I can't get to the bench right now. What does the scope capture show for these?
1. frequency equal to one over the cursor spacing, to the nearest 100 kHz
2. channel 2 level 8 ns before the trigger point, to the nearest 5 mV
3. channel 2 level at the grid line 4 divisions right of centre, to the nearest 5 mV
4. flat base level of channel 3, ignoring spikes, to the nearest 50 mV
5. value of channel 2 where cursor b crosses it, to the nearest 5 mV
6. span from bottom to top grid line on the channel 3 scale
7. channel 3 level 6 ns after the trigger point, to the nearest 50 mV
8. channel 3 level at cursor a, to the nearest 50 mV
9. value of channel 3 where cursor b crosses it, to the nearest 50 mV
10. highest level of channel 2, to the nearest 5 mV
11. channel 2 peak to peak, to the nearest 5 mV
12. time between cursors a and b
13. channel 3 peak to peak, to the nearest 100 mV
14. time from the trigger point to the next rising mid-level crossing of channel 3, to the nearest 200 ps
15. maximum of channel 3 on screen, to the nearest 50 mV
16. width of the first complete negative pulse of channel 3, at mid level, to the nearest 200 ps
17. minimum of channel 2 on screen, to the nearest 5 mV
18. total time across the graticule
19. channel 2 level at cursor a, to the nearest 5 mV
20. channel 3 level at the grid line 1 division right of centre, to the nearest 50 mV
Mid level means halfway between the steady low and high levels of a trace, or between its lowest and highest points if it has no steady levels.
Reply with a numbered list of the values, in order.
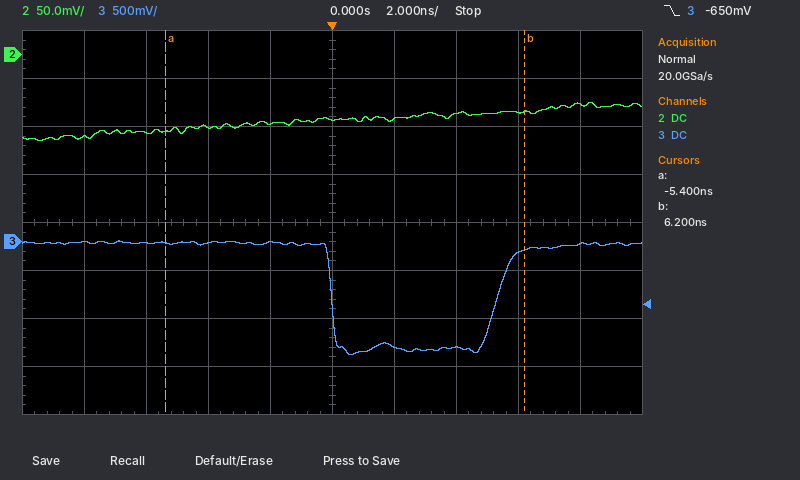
1. 86.2 MHz
2. -85 mV
3. -50 mV
4. -1.10 V
5. -60 mV
6. 4 V
7. -100 mV
8. 0 mV
9. -100 mV
10. -50 mV
11. 40 mV
12. 11.6 ns
13. 1.20 V
14. 5.4 ns
15. 0 mV
16. 5.4 ns
17. -90 mV
18. 20 ns
19. -80 mV
20. -1.10 V
